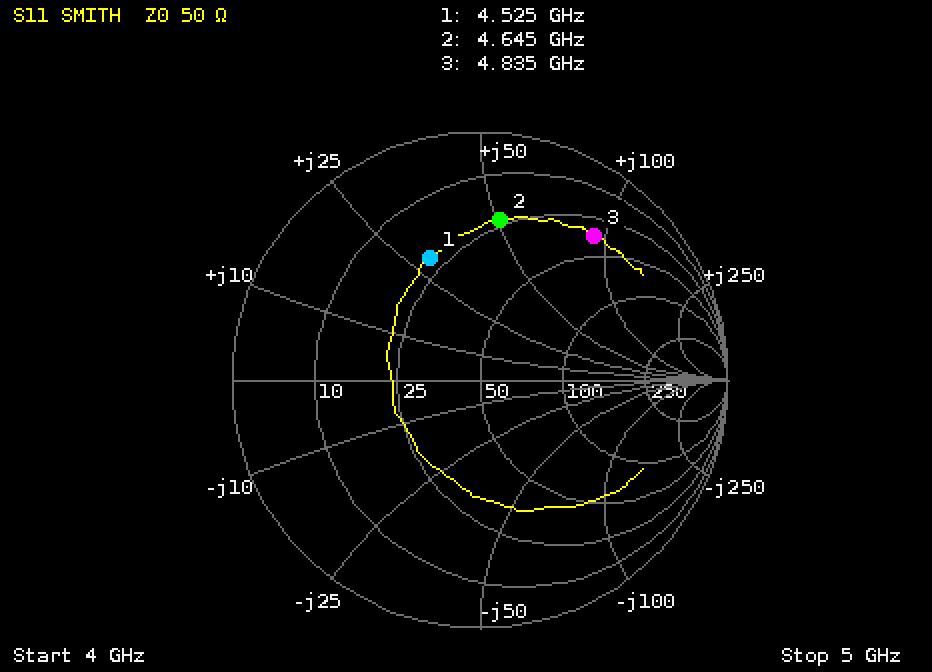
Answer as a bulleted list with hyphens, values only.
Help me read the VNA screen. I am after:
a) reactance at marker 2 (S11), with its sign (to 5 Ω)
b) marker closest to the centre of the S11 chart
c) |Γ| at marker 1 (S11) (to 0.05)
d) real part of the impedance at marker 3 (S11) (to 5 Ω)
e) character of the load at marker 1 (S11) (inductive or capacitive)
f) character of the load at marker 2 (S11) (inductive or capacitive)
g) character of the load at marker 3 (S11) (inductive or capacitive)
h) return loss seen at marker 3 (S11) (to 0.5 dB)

- +50 Ω
- marker 1
- 0.55
- 35 Ω
- inductive
- inductive
- inductive
- 2.5 dB
